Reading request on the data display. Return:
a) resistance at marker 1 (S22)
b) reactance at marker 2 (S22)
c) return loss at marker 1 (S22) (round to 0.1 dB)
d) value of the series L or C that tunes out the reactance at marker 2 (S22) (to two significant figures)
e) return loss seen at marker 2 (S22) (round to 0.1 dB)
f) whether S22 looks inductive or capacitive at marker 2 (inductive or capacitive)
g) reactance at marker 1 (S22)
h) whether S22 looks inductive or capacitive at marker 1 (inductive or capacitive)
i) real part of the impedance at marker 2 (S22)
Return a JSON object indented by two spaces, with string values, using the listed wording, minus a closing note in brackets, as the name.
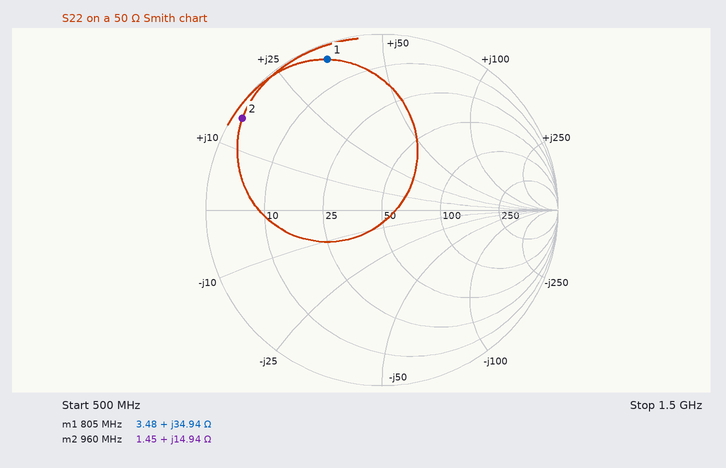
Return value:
{
  "resistance at marker 1": "3.48 Ω",
  "reactance at marker 2": "+14.94 Ω",
  "return loss at marker 1 (S22)": "0.8 dB",
  "value of the series L or C that tunes out the reactance at marker 2 (S22)": "11 pF",
  "return loss seen at marker 2 (S22)": "0.5 dB",
  "whether S22 looks inductive or capacitive at marker 2": "inductive",
  "reactance at marker 1": "+34.94 Ω",
  "whether S22 looks inductive or capacitive at marker 1": "inductive",
  "real part of the impedance at marker 2": "1.45 Ω"
}
